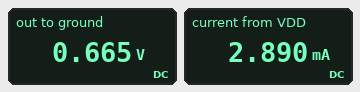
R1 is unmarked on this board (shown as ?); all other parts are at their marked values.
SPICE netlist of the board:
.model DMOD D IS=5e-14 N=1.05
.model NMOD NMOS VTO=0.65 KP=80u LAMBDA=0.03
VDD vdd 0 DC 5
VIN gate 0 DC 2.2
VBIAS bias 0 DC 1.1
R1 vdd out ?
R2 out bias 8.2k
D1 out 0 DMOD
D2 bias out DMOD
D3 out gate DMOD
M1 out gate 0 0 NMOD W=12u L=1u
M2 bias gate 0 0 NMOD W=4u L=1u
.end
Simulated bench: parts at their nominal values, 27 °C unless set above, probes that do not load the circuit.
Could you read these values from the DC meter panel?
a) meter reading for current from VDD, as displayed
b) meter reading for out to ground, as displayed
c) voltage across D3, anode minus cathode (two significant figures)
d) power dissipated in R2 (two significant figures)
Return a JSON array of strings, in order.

["2.890 mA", "0.665 V", "-1.5 V", "23 µW"]
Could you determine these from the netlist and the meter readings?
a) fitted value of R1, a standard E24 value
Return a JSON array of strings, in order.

["1.5 kΩ"]
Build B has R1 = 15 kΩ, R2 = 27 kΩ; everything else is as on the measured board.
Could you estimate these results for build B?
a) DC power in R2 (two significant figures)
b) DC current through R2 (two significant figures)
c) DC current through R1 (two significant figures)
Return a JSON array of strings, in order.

["14 µW", "23 µA", "300 µA"]
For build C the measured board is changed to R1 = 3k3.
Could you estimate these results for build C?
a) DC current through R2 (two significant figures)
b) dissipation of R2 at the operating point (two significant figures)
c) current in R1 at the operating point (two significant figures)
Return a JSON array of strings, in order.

["57 µA", "27 µW", "1.3 mA"]
